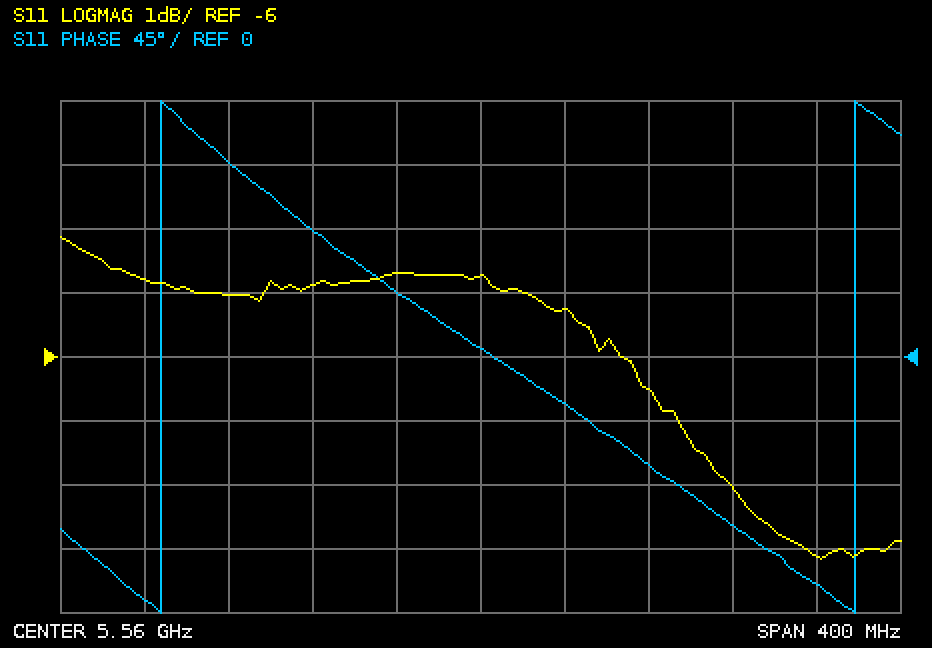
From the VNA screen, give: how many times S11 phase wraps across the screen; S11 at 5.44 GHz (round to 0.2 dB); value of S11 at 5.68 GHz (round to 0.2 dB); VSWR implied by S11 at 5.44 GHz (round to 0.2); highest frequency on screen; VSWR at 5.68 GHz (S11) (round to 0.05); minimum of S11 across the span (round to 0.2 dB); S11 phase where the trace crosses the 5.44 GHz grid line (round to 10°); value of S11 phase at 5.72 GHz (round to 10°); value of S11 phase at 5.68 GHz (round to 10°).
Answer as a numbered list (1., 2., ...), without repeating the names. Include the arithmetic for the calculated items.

1. 2
2. -5.0 dB
3. -8.0 dB
4. |Γ| = 10^(-5/20) = 0.5623; VSWR = (1 + 0.5623)/(1 − 0.5623) ≈ 3.6
5. 5.76 GHz
6. |Γ| = 10^(-8/20) = 0.3981; VSWR = (1 + 0.3981)/(1 − 0.3981) ≈ 2.32, so 2.30 to the nearest 0.05
7. -9.2 dB
8. 140°
9. -160°
10. -120°
